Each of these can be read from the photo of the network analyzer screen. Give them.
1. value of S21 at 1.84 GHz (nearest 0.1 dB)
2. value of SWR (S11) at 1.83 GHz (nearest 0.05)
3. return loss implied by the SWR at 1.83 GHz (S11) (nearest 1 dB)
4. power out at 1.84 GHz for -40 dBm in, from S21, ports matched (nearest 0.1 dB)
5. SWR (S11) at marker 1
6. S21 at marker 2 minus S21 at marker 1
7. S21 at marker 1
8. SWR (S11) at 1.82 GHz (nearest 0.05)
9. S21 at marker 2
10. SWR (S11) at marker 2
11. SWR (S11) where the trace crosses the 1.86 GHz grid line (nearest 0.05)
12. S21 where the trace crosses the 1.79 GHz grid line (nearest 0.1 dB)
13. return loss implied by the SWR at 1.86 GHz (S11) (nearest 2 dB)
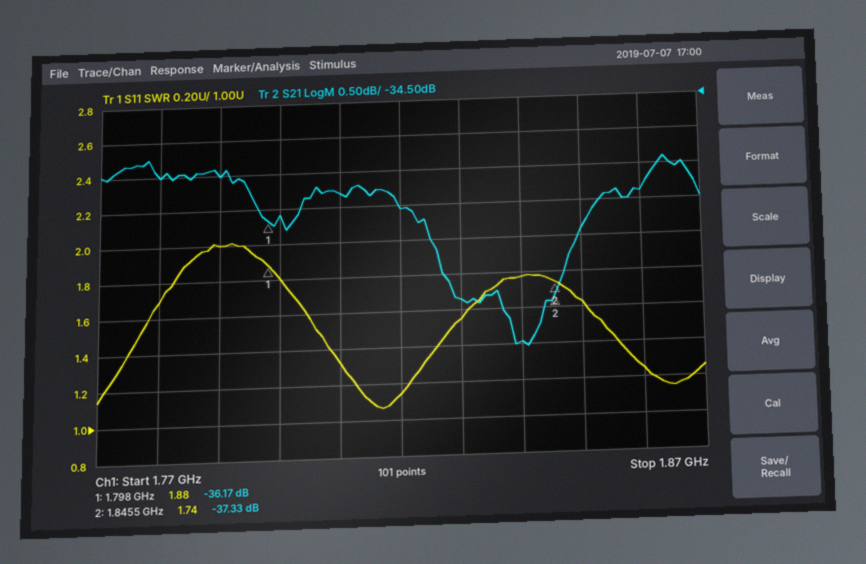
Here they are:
-38.0 dB
1.55
13 dB
-78.0 dBm
1.88
-1.16 dB
-36.17 dB
1.15
-37.33 dB
1.74
1.25
-35.5 dB
20 dB
